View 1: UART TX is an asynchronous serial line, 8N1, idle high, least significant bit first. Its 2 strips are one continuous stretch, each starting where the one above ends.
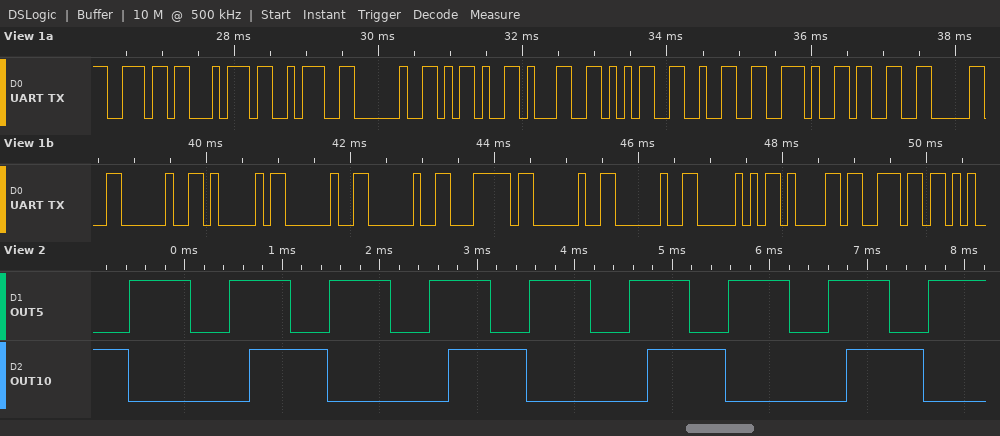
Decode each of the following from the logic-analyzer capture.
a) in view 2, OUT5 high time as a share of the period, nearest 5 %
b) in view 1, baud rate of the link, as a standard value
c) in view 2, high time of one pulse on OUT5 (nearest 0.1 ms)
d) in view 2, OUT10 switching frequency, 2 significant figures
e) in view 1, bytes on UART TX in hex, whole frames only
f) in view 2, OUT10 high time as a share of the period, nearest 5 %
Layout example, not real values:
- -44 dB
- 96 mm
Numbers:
- 60 %
- 9600 baud
- 0.6 ms
- 490 Hz
- 6E 74 3A 20 2D 31 35 32 2E 33 30 20 41 20 20 7C 20 20 50 61 6E
- 40 %
